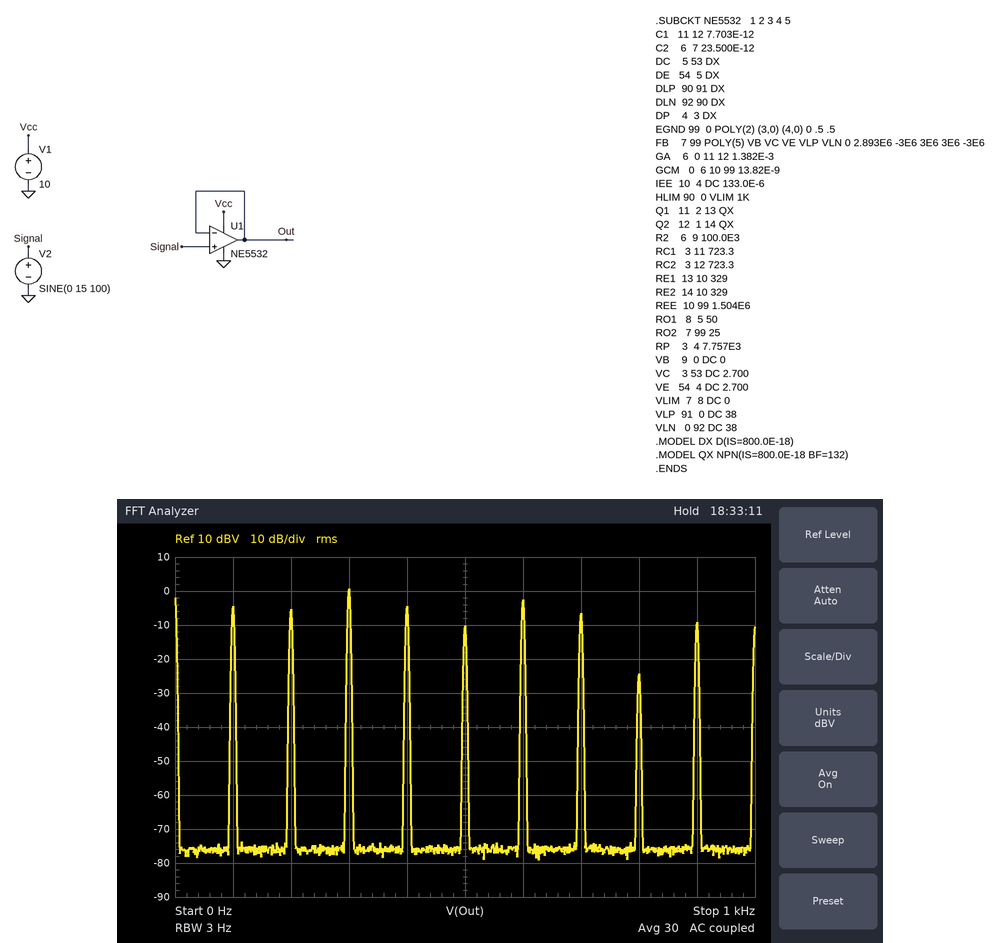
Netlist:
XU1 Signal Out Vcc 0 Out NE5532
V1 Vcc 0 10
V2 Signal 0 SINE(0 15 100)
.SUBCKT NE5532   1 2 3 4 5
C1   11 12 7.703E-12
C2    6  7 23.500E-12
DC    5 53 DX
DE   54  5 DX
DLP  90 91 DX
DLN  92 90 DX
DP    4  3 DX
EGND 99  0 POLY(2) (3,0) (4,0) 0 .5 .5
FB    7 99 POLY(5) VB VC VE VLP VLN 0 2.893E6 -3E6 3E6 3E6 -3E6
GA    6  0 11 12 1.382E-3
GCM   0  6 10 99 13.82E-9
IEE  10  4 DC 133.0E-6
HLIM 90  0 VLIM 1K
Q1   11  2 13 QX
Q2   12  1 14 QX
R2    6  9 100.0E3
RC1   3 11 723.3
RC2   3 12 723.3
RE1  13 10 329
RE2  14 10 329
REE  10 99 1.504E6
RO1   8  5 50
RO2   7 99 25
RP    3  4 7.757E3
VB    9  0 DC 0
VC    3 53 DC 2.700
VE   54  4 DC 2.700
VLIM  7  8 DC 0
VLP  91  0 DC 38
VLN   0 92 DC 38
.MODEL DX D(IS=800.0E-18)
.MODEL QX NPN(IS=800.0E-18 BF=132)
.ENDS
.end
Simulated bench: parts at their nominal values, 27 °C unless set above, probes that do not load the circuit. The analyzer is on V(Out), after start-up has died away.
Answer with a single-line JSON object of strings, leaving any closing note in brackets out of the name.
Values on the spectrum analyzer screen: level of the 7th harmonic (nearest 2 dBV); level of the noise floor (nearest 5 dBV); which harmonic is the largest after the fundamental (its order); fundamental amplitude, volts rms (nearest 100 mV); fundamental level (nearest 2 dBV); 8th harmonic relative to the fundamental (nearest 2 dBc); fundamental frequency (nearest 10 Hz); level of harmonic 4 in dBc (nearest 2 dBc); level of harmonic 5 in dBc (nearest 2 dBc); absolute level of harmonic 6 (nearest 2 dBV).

{"level of the 7th harmonic": "-6 dBV", "level of the noise floor": "-75 dBV", "which harmonic is the largest after the fundamental": "3", "fundamental amplitude, volts rms": "600 mV", "fundamental level": "-4 dBV", "8th harmonic relative to the fundamental": "-20 dBc", "fundamental frequency": "100 Hz", "level of harmonic 4 in dBc": "0 dBc", "level of harmonic 5 in dBc": "-6 dBc", "absolute level of harmonic 6": "-2 dBV"}
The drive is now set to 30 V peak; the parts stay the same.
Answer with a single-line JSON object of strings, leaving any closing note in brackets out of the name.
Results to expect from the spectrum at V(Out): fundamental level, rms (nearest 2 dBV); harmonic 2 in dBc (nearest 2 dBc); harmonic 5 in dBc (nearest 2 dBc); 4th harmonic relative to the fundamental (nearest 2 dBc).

{"fundamental level, rms": "-22 dBV", "harmonic 2 in dBc": "16 dBc", "harmonic 5 in dBc": "16 dBc", "4th harmonic relative to the fundamental": "10 dBc"}
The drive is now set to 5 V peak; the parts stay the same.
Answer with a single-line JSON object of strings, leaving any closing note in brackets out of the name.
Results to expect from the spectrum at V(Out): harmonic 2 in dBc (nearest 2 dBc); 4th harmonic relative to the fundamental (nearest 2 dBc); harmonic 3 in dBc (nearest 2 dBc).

{"harmonic 2 in dBc": "-4 dBc", "4th harmonic relative to the fundamental": "-60 dBc", "harmonic 3 in dBc": "-12 dBc"}
